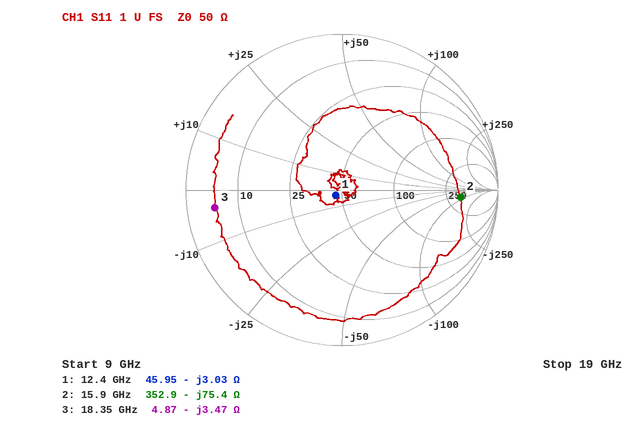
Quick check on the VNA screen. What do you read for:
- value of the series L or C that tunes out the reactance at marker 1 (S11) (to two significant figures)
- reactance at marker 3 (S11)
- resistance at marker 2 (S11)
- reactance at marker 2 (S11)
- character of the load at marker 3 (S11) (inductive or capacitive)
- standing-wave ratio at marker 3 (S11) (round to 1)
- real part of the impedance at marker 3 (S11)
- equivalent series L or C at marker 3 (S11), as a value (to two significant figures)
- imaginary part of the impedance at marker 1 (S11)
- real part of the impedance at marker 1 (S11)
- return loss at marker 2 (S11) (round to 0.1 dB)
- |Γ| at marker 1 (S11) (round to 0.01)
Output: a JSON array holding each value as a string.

["39 pH", "-3.47 Ω", "352.9 Ω", "-75.4 Ω", "capacitive", "10", "4.87 Ω", "2.5 pF", "-3.03 Ω", "45.95 Ω", "2.4 dB", "0.05"]
